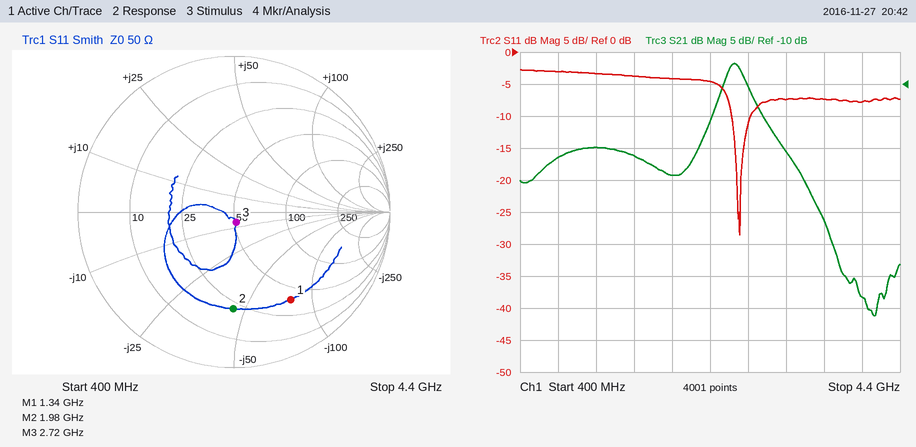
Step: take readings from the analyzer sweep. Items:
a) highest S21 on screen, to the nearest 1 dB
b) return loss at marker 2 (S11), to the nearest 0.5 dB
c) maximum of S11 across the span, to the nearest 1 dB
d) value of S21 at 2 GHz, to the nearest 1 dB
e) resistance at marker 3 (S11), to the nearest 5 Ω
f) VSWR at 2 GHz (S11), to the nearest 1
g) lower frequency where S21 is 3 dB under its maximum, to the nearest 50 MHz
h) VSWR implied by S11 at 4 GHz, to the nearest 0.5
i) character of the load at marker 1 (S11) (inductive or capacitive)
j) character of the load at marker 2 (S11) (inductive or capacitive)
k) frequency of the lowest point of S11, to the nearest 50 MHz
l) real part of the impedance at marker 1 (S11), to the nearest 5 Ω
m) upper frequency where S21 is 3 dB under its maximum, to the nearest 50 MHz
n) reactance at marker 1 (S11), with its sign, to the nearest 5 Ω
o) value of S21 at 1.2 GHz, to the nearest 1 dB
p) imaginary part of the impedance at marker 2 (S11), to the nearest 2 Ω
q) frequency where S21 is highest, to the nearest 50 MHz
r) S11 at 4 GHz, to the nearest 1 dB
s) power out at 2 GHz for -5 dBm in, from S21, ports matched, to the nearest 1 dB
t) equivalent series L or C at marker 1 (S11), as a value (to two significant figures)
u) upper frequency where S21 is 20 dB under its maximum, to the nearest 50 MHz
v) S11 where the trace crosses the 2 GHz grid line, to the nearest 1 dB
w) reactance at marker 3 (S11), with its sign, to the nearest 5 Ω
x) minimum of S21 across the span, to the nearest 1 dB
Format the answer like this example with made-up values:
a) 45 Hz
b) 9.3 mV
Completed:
a) -7 dB
b) 4.0 dB
c) -3 dB
d) -24 dB
e) 50 Ω
f) 4
g) 2.55 GHz
h) 2.5
i) capacitive
j) capacitive
k) 2.70 GHz
l) 40 Ω
m) 2.80 GHz
n) -80 Ω
o) -20 dB
p) -44 Ω
q) 2.65 GHz
r) -8 dB
s) -29 dBm
t) 1.5 pF
u) 3.45 GHz
v) -4 dB
w) -5 Ω
x) -46 dB
